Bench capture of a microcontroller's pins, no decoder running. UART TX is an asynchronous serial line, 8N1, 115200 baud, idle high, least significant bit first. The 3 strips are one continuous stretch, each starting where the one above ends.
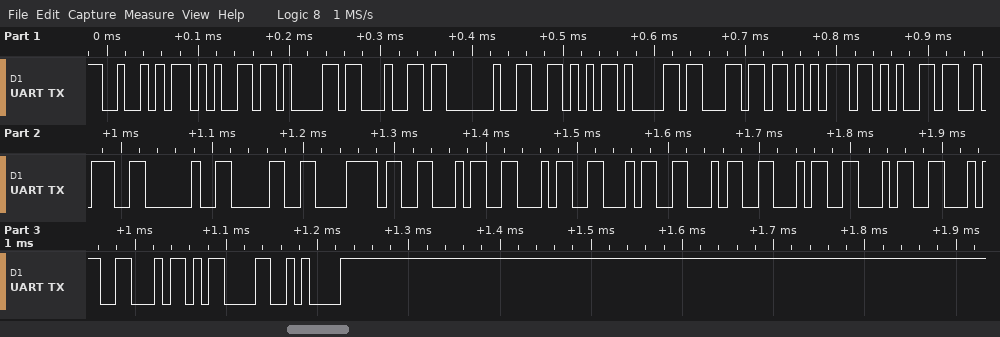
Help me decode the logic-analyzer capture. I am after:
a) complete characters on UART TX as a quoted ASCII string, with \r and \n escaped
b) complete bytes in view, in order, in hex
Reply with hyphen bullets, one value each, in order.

- "Read Value: 0xFFFFFFFF\r\n"
- 52 65 61 64 20 56 61 6C 75 65 3A 20 30 78 46 46 46 46 46 46 46 46 0D 0A
